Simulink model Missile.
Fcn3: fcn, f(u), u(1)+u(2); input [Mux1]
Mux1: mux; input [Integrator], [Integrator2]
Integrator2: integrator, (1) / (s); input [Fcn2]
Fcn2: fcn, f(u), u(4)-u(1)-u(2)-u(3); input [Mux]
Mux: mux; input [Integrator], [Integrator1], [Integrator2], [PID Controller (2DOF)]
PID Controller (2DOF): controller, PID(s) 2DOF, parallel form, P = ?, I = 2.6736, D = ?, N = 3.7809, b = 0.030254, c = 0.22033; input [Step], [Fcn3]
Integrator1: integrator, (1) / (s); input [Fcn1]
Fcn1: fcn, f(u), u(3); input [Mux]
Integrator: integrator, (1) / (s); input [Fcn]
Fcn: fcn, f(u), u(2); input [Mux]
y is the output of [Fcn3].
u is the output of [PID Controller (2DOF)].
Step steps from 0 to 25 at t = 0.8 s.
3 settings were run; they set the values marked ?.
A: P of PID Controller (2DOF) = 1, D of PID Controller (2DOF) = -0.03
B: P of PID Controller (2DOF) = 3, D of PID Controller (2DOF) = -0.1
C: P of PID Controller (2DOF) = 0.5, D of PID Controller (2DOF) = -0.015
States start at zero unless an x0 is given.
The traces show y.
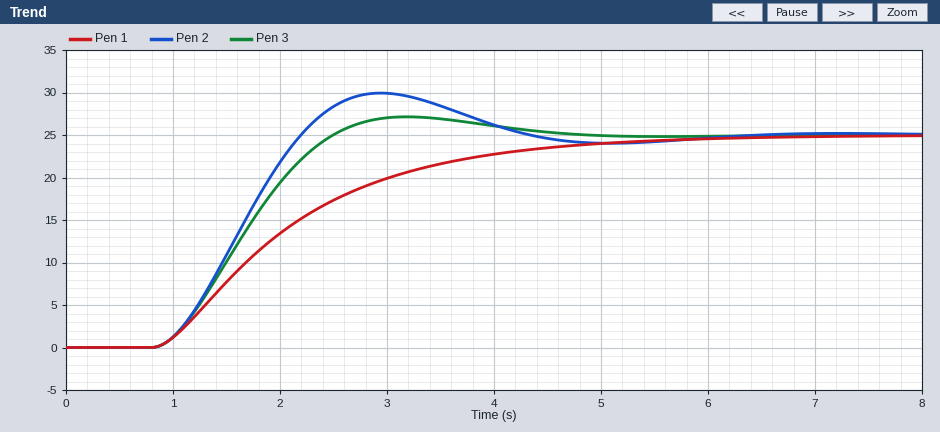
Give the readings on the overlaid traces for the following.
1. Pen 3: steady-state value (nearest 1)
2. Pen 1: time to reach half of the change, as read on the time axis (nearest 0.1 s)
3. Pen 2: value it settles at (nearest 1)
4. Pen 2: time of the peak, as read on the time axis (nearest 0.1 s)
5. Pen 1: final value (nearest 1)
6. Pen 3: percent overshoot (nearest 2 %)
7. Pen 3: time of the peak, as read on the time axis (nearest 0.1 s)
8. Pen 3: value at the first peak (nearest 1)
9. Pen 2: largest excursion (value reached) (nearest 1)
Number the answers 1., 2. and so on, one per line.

1. 25
2. 1.9 s
3. 25
4. 2.9 s
5. 25
6. 8 %
7. 3.2 s
8. 27
9. 30
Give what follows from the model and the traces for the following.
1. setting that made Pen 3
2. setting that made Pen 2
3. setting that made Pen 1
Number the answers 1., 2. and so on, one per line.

1. A
2. C
3. B
